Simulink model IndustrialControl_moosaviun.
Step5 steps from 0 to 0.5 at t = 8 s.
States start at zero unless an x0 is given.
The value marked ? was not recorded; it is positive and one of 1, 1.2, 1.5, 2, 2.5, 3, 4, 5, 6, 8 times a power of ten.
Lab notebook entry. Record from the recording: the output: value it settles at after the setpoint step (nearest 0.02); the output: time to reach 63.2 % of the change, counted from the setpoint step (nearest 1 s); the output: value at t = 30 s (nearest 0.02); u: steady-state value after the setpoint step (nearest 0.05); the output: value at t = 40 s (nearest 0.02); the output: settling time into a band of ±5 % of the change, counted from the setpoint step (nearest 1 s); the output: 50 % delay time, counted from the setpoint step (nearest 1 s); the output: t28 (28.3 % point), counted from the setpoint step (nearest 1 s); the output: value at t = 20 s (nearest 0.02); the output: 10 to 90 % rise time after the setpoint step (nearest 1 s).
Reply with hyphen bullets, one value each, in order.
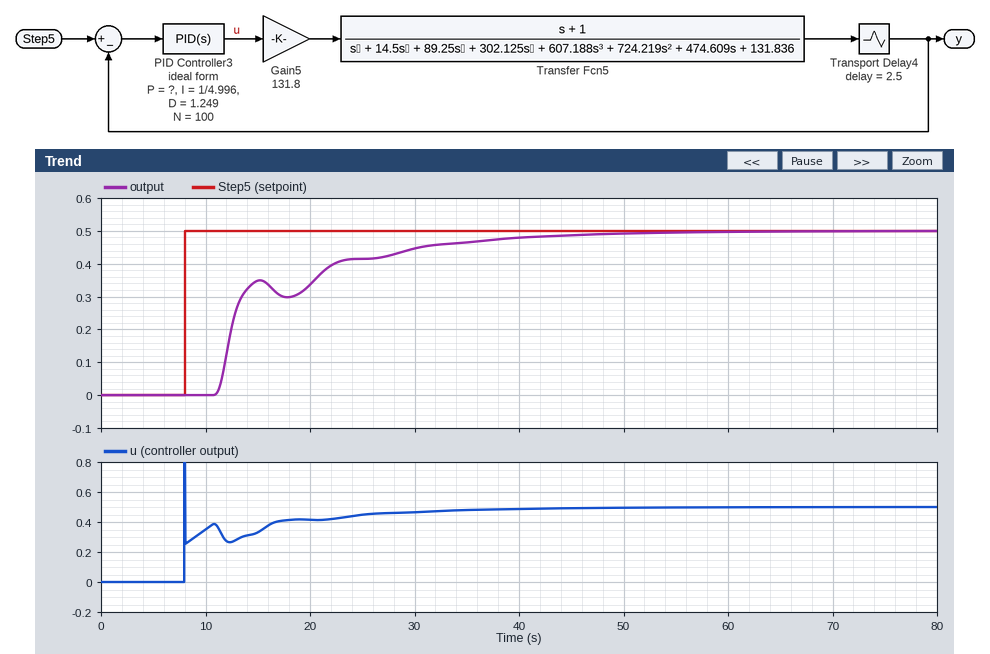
- 0.50
- 6 s
- 0.44
- 0.50
- 0.48
- 30 s
- 5 s
- 4 s
- 0.34
- 19 s
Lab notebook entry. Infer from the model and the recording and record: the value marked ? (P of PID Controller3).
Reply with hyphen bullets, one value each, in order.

- 0.5
